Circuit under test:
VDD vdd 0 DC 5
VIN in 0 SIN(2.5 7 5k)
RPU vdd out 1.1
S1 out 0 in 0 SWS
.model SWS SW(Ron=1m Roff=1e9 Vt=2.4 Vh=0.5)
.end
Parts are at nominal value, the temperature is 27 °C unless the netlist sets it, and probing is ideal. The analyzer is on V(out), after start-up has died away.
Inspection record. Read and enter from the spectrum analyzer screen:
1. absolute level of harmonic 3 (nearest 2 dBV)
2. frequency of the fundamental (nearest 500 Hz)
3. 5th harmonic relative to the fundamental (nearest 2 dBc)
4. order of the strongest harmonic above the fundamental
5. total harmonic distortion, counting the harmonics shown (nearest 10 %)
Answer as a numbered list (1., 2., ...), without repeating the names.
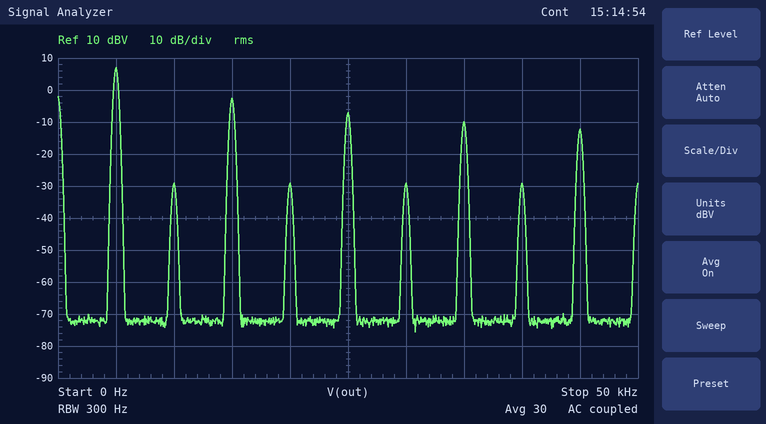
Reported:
1. -2 dBV
2. 5.0 kHz
3. -14 dBc
4. 3
5. 40 %
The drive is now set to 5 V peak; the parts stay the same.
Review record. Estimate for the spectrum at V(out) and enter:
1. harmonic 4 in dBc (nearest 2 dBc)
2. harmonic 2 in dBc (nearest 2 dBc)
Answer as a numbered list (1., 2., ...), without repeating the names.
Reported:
1. -34 dBc
2. -34 dBc
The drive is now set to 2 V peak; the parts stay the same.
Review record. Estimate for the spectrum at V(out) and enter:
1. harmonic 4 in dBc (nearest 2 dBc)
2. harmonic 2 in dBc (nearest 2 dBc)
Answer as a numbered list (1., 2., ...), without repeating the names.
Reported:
1. -26 dBc
2. -26 dBc
